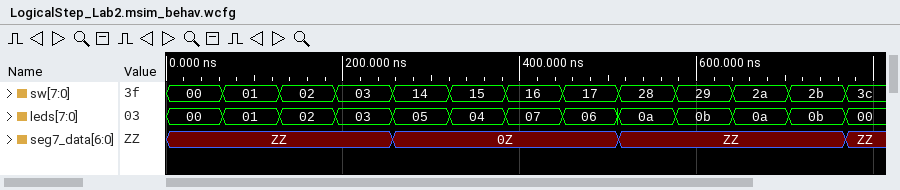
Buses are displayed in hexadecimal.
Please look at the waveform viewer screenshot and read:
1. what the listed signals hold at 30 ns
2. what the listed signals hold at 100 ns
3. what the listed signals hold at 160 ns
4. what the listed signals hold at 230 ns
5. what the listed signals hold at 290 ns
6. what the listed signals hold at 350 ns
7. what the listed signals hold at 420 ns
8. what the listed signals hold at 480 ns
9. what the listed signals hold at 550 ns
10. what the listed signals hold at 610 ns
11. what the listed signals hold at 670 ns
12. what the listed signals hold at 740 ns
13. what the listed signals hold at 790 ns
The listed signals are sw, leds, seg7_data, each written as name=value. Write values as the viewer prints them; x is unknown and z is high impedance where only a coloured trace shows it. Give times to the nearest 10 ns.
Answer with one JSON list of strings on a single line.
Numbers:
["sw=00, leds=00, seg7_data=ZZ", "sw=01, leds=01, seg7_data=ZZ", "sw=02, leds=02, seg7_data=ZZ", "sw=03, leds=03, seg7_data=ZZ", "sw=14, leds=05, seg7_data=0Z", "sw=15, leds=04, seg7_data=0Z", "sw=16, leds=07, seg7_data=0Z", "sw=17, leds=06, seg7_data=0Z", "sw=28, leds=0a, seg7_data=ZZ", "sw=29, leds=0b, seg7_data=ZZ", "sw=2a, leds=0a, seg7_data=ZZ", "sw=2b, leds=0b, seg7_data=ZZ", "sw=3c, leds=00, seg7_data=ZZ"]
